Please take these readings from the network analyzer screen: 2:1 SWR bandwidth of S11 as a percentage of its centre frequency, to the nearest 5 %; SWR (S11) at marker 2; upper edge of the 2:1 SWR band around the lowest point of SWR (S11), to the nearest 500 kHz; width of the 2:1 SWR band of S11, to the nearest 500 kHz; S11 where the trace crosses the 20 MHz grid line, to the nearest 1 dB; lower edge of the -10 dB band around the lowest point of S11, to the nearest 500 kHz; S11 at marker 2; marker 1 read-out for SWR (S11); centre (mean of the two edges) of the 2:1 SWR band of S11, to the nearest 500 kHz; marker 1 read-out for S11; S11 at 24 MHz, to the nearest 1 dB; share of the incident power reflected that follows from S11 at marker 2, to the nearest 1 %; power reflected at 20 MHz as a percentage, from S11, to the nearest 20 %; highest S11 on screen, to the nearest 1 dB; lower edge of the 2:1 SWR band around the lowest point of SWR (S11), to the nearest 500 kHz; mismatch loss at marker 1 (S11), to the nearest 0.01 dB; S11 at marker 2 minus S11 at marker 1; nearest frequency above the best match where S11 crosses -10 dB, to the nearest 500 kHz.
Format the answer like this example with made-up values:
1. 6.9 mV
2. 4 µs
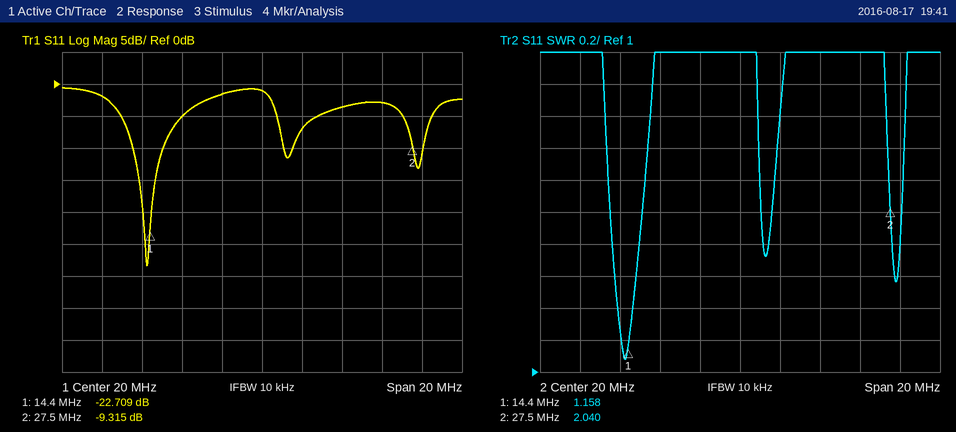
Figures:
1. 10 %
2. 2.040
3. 15.0 MHz
4. 1.5 MHz
5. -1 dB
6. 13.5 MHz
7. -9.315 dB
8. 1.158
9. 14.5 MHz
10. -22.709 dB
11. -4 dB
12. 12 %
13. 80 %
14. -1 dB
15. 13.5 MHz
16. 0.02 dB
17. 13.394 dB
18. 15.0 MHz
